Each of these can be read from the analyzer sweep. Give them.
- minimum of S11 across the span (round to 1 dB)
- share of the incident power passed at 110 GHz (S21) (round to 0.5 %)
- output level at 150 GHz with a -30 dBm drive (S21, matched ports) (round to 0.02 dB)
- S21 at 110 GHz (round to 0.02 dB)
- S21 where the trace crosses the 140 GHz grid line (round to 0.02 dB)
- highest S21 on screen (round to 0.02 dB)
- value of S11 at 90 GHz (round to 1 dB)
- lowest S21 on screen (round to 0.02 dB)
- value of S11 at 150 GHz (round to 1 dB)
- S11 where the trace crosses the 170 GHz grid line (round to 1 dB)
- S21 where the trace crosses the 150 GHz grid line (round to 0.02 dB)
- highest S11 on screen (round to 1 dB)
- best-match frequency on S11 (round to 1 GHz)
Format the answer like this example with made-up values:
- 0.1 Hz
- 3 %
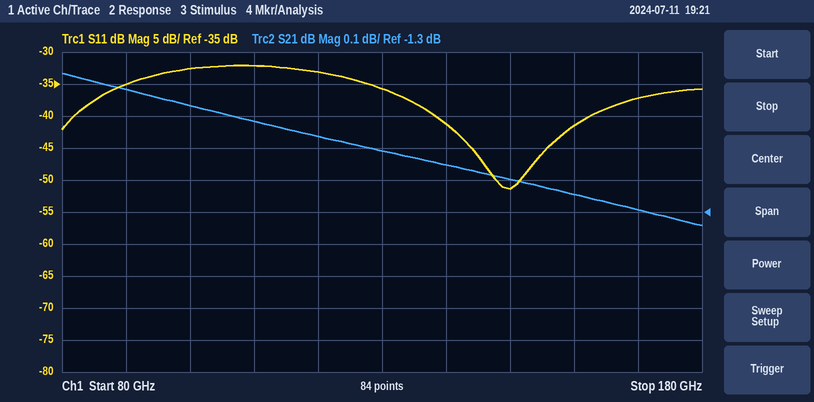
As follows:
- -51 dB
- 79.0 %
- -31.20 dBm
- -1.02 dB
- -1.16 dB
- -0.86 dB
- -35 dB
- -1.34 dB
- -51 dB
- -37 dB
- -1.20 dB
- -32 dB
- 150 GHz
